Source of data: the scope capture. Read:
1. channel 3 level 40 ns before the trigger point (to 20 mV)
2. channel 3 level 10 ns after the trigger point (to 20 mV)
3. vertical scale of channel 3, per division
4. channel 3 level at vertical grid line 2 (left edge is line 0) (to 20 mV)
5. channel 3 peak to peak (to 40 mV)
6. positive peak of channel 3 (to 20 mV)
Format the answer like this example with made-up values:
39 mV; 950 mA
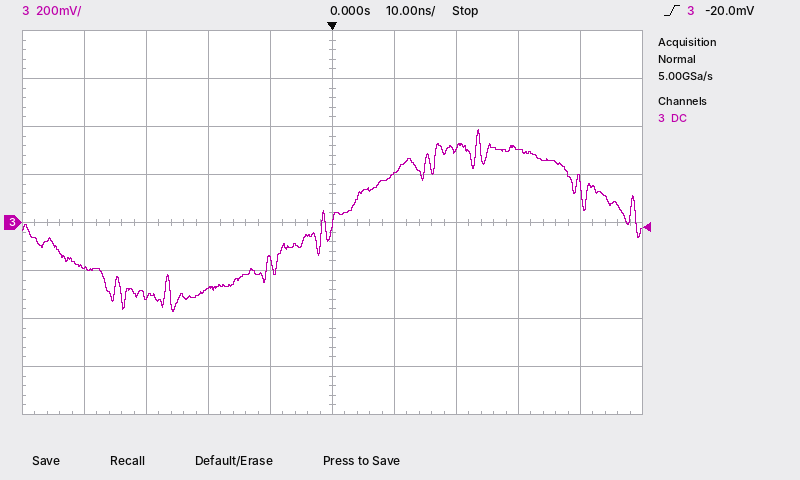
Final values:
-180 mV; 200 mV; 200 mV; -300 mV; 760 mV; 380 mV
